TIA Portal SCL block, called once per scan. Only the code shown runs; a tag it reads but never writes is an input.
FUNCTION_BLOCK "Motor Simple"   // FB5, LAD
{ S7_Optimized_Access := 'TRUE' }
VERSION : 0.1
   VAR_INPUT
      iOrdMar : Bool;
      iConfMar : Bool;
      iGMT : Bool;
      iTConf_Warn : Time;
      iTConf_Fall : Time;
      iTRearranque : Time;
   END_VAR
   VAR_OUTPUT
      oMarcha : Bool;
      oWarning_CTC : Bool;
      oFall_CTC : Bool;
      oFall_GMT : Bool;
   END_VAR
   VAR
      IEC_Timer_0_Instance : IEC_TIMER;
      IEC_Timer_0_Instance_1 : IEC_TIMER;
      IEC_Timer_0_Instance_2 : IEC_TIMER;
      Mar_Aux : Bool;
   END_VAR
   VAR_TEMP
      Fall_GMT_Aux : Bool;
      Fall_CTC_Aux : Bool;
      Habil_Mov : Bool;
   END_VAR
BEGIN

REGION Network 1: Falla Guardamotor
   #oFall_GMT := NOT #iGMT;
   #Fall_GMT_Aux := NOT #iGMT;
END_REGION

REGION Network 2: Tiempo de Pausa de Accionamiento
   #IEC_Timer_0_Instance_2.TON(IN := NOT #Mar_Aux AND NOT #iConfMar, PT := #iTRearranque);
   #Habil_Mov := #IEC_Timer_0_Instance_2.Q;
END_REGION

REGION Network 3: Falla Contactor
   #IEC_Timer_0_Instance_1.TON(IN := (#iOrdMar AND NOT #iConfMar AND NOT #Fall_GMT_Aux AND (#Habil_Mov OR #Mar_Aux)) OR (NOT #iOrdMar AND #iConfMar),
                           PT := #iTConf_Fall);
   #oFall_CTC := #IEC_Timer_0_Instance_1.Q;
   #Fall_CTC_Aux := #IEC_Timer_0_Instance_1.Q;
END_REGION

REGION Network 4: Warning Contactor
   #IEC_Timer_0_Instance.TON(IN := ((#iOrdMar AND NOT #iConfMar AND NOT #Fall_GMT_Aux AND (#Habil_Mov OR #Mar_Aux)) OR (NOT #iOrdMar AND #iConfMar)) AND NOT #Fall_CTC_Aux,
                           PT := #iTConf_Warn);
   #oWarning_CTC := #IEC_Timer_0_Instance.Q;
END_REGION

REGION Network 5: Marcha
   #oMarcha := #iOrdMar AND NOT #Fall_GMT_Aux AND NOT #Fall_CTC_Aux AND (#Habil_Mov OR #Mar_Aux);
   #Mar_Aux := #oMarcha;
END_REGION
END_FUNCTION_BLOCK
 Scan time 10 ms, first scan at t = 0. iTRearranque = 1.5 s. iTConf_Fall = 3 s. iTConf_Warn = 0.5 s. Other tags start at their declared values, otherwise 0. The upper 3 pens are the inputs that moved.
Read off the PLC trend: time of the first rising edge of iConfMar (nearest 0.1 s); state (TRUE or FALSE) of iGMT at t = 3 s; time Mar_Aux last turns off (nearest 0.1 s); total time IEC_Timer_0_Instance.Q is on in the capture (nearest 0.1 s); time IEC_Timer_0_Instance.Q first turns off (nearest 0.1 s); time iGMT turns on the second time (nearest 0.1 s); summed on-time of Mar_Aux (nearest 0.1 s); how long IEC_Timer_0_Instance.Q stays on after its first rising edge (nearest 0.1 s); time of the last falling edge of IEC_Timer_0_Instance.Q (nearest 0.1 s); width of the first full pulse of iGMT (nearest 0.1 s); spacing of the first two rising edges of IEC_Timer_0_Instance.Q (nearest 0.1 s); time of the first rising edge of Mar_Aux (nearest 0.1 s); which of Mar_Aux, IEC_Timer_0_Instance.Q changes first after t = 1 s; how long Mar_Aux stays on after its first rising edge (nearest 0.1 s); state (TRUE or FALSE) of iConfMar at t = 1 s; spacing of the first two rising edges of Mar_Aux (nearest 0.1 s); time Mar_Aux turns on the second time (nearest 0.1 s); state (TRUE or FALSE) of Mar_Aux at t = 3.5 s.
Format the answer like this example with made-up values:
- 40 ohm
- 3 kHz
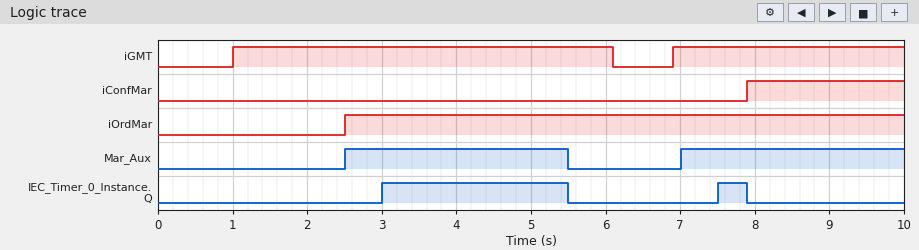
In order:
- 7.9 s
- TRUE
- 5.5 s
- 2.9 s
- 5.5 s
- 6.9 s
- 6.0 s
- 2.5 s
- 7.9 s
- 5.1 s
- 4.5 s
- 2.5 s
- Mar_Aux
- 3.0 s
- FALSE
- 4.5 s
- 7.0 s
- TRUE
